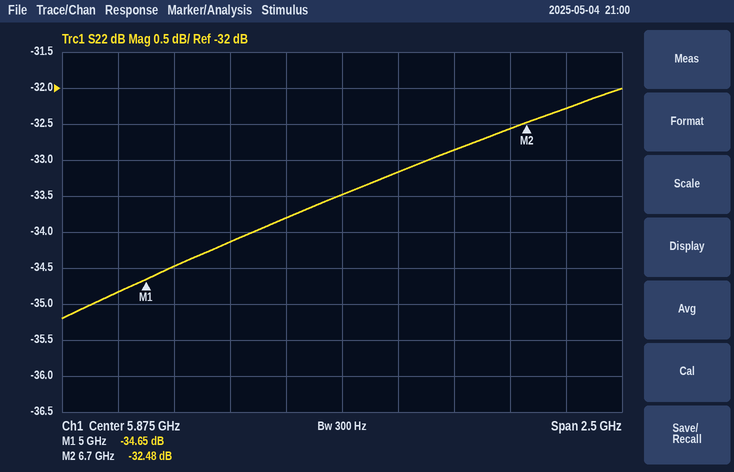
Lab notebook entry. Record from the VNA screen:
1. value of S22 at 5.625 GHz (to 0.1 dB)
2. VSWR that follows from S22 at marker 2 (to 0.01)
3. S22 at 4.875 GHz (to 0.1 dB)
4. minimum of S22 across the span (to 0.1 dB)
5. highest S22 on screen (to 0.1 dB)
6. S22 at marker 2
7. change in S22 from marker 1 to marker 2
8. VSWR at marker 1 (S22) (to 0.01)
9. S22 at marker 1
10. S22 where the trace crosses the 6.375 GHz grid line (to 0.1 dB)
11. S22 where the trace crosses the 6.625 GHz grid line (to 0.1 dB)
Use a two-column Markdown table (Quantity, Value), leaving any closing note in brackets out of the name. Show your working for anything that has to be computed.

| Quantity | Value |
|---|---|
| value of S22 at 5.625 GHz | -33.8 dB |
| VSWR that follows from S22 at marker 2 | (1 + 0.0238)/(1 − 0.0238) ≈ 1.05 |
| S22 at 4.875 GHz | -34.8 dB |
| minimum of S22 across the span | -35.2 dB |
| highest S22 on screen | -32.0 dB |
| S22 at marker 2 | -32.48 dB |
| change in S22 from marker 1 to marker 2 | -32.48 − (-34.65) = 2.17 dB |
| VSWR at marker 1 (S22) | (1 + 0.0185)/(1 − 0.0185) ≈ 1.04 |
| S22 at marker 1 | -34.65 dB |
| S22 where the trace crosses the 6.375 GHz grid line | -32.9 dB |
| S22 where the trace crosses the 6.625 GHz grid line | -32.6 dB |
